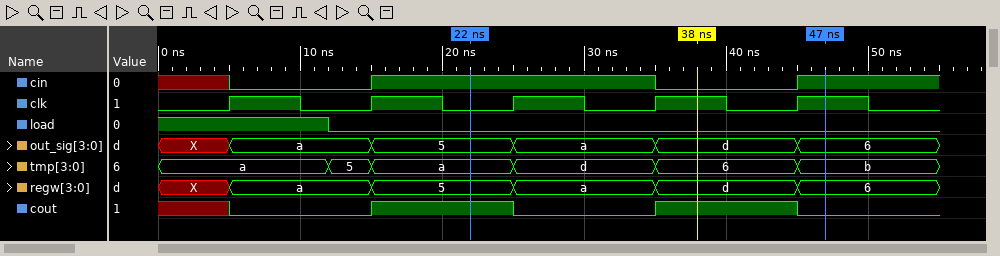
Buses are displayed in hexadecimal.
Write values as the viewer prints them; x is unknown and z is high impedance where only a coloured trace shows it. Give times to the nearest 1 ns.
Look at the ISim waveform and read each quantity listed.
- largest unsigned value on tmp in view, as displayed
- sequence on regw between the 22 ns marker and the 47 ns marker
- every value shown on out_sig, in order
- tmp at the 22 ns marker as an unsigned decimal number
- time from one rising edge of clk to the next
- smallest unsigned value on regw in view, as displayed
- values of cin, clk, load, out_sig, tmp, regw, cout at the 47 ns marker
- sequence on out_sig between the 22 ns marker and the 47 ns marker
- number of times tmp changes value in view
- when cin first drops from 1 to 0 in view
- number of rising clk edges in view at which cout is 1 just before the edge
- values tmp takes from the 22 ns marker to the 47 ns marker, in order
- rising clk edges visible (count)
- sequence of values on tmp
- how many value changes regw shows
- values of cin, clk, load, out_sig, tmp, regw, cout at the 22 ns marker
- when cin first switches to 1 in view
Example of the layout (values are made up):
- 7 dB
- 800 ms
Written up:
- d
- 5, a, d, 6
- X, a, 5, a, d, 6
- 10
- 10 ns
- 5
- cin=1, clk=1, load=0, out_sig=6, tmp=b, regw=6, cout=0
- 5, a, d, 6
- 5
- 35 ns
- 2
- a, d, 6, b
- 5
- a, 5, a, d, 6, b
- 5
- cin=1, clk=0, load=0, out_sig=5, tmp=a, regw=5, cout=1
- 15 ns
